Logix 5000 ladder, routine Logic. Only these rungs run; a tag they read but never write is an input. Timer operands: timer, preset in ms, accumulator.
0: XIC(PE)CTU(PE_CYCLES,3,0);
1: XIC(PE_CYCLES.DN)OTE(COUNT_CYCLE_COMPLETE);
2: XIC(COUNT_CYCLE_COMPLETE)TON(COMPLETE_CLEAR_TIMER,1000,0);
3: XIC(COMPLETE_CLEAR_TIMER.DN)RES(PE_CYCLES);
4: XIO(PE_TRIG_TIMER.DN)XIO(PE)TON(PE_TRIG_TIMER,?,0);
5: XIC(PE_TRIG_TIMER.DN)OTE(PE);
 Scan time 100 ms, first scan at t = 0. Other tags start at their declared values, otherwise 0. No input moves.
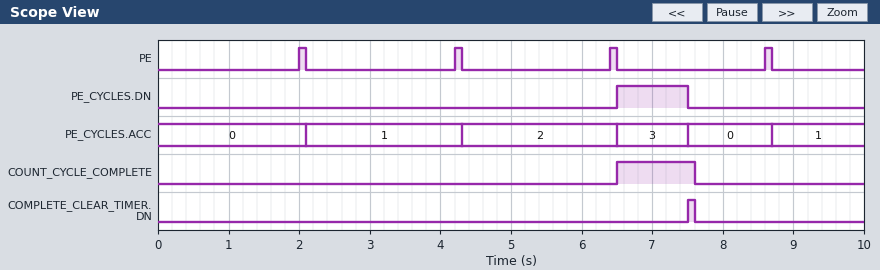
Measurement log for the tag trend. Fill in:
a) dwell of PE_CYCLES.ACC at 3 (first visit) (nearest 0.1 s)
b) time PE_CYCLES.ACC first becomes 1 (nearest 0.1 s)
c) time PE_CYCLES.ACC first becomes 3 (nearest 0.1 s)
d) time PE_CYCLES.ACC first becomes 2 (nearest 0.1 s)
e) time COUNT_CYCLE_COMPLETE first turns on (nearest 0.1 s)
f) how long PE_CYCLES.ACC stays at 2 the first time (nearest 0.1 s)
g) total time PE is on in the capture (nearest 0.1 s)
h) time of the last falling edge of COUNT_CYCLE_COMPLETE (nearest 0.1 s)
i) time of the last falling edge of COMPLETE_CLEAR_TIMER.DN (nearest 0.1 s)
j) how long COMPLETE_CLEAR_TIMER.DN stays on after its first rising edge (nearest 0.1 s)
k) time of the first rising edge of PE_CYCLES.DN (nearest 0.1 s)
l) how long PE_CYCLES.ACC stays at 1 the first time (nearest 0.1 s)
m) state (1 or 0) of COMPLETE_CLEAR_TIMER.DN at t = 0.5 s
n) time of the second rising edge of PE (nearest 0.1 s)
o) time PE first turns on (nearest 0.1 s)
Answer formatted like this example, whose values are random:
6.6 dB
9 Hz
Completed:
1.0 s
2.1 s
6.5 s
4.3 s
6.5 s
2.2 s
0.4 s
7.6 s
7.6 s
0.1 s
6.5 s
2.2 s
0
4.2 s
2.0 s
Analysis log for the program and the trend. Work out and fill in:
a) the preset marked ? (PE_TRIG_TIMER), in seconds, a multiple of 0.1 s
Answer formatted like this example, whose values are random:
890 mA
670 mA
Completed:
2.0 s
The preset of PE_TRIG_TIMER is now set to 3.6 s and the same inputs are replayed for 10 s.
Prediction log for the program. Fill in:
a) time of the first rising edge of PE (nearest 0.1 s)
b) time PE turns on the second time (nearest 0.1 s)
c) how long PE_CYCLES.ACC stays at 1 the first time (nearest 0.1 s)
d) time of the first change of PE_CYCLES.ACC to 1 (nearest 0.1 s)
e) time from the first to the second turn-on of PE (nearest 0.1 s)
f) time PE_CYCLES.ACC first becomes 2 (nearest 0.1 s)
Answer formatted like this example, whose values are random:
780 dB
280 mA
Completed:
3.6 s
7.4 s
3.8 s
3.7 s
3.8 s
7.5 s
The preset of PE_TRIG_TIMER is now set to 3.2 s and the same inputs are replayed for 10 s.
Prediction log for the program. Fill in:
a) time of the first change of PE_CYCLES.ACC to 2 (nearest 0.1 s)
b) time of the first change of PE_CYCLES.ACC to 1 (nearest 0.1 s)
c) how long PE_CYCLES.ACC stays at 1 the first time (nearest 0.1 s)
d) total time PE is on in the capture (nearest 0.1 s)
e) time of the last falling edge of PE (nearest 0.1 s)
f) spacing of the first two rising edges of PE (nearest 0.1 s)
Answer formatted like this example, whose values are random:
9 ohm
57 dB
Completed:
6.7 s
3.3 s
3.4 s
0.2 s
6.7 s
3.4 s
